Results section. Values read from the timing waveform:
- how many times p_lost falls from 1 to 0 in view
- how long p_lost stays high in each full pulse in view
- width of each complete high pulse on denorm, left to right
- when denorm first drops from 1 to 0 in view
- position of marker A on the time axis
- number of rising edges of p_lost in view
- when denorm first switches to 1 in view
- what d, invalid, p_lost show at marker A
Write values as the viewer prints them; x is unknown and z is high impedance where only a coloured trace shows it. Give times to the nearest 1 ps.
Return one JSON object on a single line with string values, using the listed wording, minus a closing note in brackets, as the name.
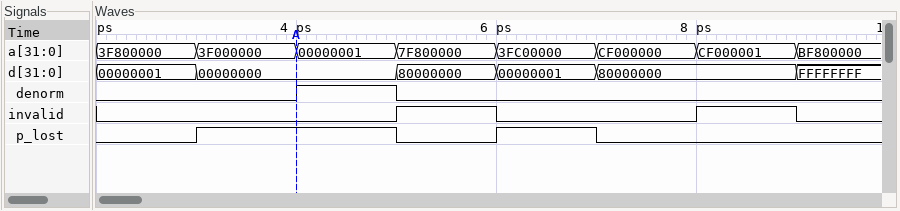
{"how many times p_lost falls from 1 to 0 in view": "2", "how long p_lost stays high in each full pulse in view": "2 ps, 1 ps", "width of each complete high pulse on denorm, left to right": "1 ps", "when denorm first drops from 1 to 0 in view": "5 ps", "position of marker A on the time axis": "4 ps", "number of rising edges of p_lost in view": "2", "when denorm first switches to 1 in view": "4 ps", "what d, invalid, p_lost show at marker A": "d=00000000, invalid=0, p_lost=1"}
